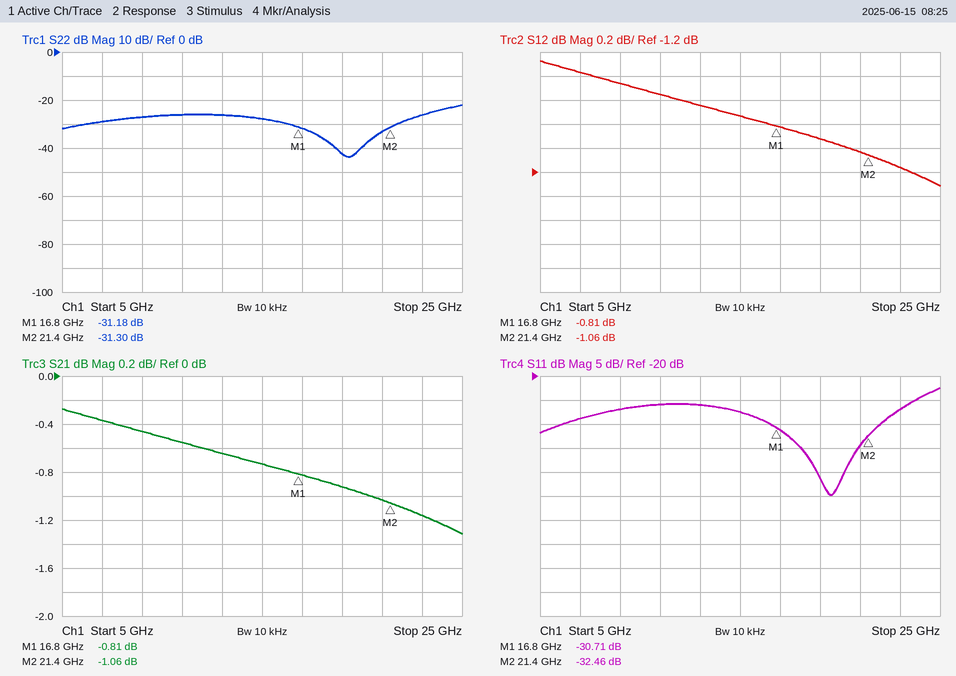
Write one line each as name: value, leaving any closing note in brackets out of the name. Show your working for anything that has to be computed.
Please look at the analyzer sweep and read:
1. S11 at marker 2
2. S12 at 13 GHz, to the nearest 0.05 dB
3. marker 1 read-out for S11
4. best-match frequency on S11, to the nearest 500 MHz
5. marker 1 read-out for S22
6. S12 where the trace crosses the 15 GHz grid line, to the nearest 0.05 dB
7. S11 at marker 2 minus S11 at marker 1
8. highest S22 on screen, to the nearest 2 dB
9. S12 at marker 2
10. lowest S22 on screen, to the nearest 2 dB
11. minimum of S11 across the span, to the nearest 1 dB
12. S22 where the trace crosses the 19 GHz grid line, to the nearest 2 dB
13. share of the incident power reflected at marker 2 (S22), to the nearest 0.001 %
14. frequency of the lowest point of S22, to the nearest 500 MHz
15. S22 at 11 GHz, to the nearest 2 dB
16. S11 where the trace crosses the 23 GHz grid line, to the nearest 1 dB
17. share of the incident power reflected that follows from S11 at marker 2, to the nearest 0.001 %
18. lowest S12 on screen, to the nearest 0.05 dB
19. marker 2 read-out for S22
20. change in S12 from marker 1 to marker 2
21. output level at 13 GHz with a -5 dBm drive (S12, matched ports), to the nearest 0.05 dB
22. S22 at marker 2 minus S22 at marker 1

S11 at marker 2: -32.46 dB
S12 at 13 GHz, to the nearest 0.05 dB: -0.65 dB
marker 1 read-out for S11: -30.71 dB
best-match frequency on S11, to the nearest 500 MHz: 19.5 GHz
marker 1 read-out for S22: -31.18 dB
S12 where the trace crosses the 15 GHz grid line, to the nearest 0.05 dB: -0.75 dB
S11 at marker 2 minus S11 at marker 1: -32.46 − (-30.71) = -1.75 dB
highest S22 on screen, to the nearest 2 dB: -22 dB
S12 at marker 2: -1.06 dB
lowest S22 on screen, to the nearest 2 dB: -44 dB
minimum of S11 across the span, to the nearest 1 dB: -45 dB
S22 where the trace crosses the 19 GHz grid line, to the nearest 2 dB: -42 dB
share of the incident power reflected at marker 2 (S22), to the nearest 0.001 %: 10^(-31.3/10) ≈ 0.074 %
frequency of the lowest point of S22, to the nearest 500 MHz: 19.5 GHz
S22 at 11 GHz, to the nearest 2 dB: -26 dB
S11 where the trace crosses the 23 GHz grid line, to the nearest 1 dB: -27 dB
share of the incident power reflected that follows from S11 at marker 2, to the nearest 0.001 %: 10^(-32.46/10) ≈ 0.057 %
lowest S12 on screen, to the nearest 0.05 dB: -1.30 dB
marker 2 read-out for S22: -31.30 dB
change in S12 from marker 1 to marker 2: -1.06 − (-0.81) = -0.25 dB
output level at 13 GHz with a -5 dBm drive (S12, matched ports), to the nearest 0.05 dB: -5 dBm + (-0.65 dB) = -5.65 dBm
S22 at marker 2 minus S22 at marker 1: -31.3 − (-31.18) = -0.12 dB
